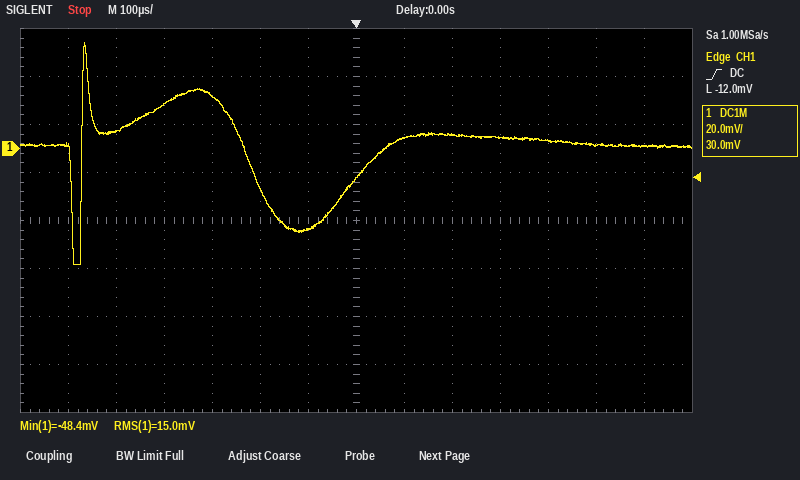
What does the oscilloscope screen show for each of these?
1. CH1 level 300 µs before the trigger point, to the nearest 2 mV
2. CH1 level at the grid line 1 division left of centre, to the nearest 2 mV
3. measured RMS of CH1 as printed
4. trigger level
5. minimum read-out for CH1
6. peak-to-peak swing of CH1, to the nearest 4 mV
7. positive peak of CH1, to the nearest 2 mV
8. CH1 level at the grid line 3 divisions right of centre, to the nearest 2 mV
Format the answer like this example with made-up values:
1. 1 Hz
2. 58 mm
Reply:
1. 22 mV
2. -34 mV
3. 15.0 mV
4. -12.0 mV
5. -48.4 mV
6. 92 mV
7. 44 mV
8. 4 mV
